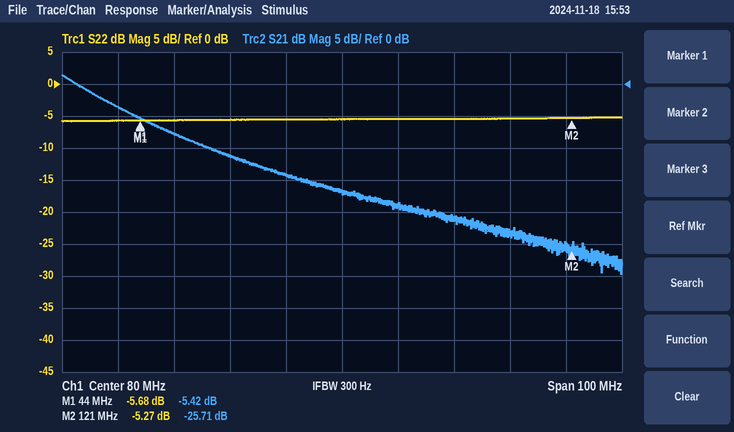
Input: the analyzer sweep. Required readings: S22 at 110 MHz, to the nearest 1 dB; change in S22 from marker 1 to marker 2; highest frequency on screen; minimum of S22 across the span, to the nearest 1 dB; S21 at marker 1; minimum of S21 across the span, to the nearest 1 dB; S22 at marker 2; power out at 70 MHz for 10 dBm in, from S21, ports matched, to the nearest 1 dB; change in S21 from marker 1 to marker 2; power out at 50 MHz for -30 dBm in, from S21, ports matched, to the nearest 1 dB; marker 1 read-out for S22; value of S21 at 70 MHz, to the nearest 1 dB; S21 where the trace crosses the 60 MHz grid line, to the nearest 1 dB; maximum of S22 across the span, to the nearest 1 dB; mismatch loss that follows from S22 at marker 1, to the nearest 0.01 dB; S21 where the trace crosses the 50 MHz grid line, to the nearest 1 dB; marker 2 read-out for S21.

-5 dB
0.41 dB
130 MHz
-6 dB
-5.42 dB
-30 dB
-5.27 dB
-4 dBm
-20.29 dB
-38 dBm
-5.68 dB
-14 dB
-11 dB
-5 dB
1.37 dB
-8 dB
-25.71 dB
